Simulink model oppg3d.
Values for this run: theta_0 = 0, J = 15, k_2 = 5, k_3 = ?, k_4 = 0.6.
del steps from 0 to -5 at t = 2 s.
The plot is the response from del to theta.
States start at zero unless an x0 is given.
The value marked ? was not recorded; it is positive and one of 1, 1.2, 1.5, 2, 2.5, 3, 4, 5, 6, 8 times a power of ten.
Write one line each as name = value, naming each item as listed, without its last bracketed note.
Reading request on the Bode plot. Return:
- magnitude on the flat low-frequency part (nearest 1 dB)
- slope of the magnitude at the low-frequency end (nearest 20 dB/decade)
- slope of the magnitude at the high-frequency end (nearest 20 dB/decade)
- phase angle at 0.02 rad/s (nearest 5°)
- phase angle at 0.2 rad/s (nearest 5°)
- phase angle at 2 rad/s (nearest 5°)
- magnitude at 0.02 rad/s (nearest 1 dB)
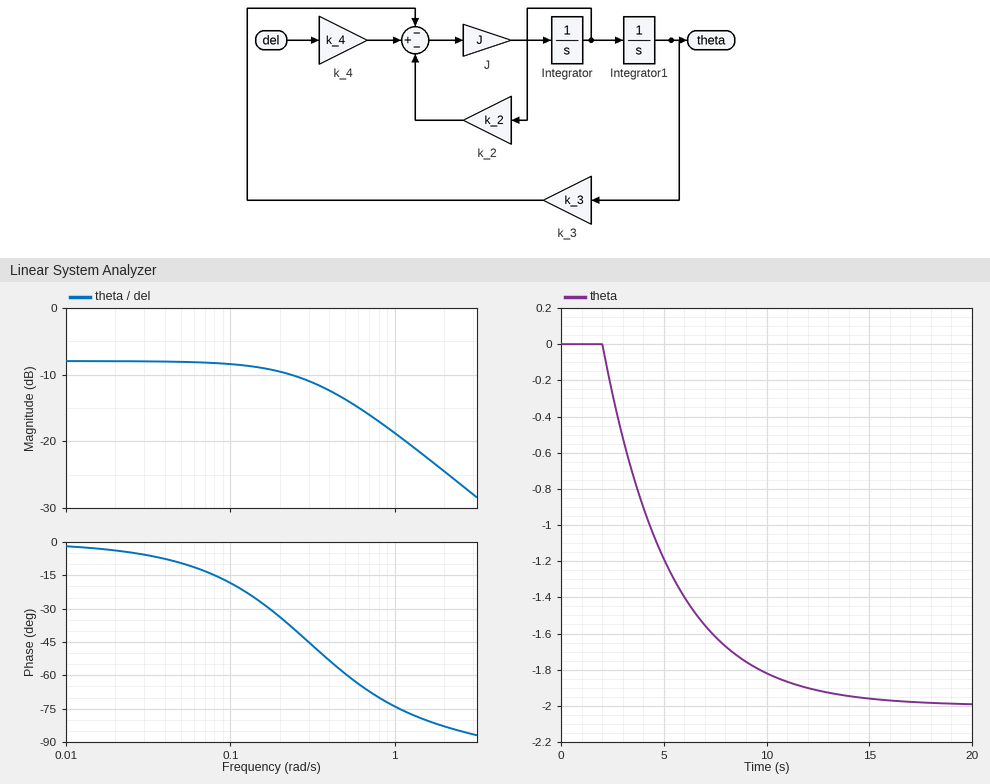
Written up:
magnitude on the flat low-frequency part = -8 dB
slope of the magnitude at the low-frequency end = 0 dB/decade
slope of the magnitude at the high-frequency end = -20 dB/decade
phase angle at 0.02 rad/s = -5°
phase angle at 0.2 rad/s = -35°
phase angle at 2 rad/s = -85°
magnitude at 0.02 rad/s = -8 dB
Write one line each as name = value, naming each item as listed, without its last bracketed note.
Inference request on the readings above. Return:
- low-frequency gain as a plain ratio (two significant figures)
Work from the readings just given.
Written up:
low-frequency gain as a plain ratio = 0.40
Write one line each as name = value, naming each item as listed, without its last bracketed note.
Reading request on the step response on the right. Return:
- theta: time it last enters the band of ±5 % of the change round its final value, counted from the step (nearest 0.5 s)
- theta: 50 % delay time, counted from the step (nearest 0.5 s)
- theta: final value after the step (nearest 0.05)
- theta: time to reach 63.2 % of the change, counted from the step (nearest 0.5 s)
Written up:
theta: time it last enters the band of ±5 % of the change round its final value, counted from the step = 10.0 s
theta: 50 % delay time, counted from the step = 2.5 s
theta: final value after the step = -2.00
theta: time to reach 63.2 % of the change, counted from the step = 3.5 s
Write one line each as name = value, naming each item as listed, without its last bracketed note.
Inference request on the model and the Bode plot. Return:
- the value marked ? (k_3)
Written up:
the value marked ? = 1.5
